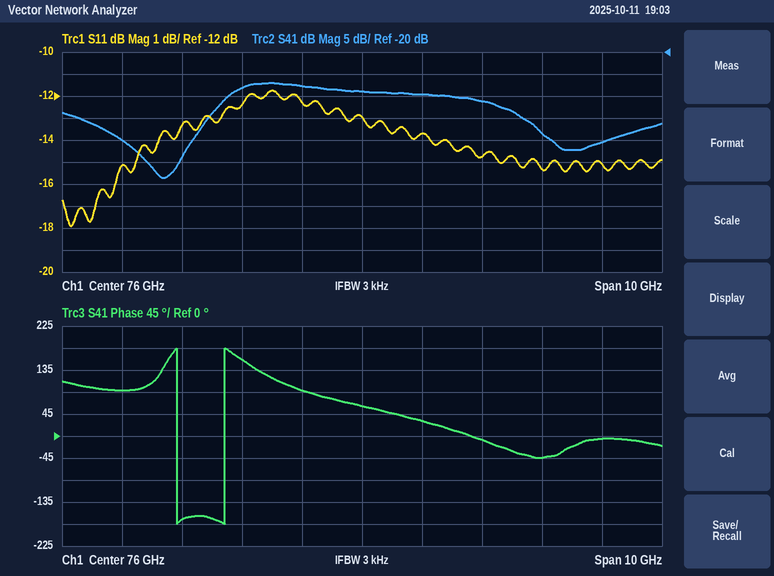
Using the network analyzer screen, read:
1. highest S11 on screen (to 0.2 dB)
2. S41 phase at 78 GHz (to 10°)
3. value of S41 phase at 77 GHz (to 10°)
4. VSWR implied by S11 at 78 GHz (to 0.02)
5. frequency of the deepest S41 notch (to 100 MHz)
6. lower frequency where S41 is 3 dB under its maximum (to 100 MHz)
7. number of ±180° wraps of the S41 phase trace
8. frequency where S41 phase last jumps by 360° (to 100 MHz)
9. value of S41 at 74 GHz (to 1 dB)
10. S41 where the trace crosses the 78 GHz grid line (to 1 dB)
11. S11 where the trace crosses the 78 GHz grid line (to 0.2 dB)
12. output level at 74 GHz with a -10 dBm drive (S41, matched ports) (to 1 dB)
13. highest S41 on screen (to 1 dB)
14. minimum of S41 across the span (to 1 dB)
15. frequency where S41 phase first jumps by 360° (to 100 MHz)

-11.8 dB
-10°
30°
1.44
72.7 GHz
73.8 GHz
2
73.7 GHz
-28 dB
-31 dB
-14.8 dB
-38 dBm
-27 dB
-49 dB
72.9 GHz
